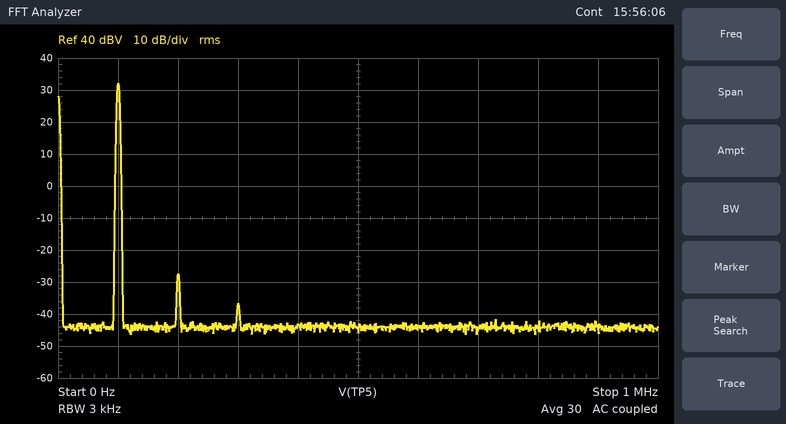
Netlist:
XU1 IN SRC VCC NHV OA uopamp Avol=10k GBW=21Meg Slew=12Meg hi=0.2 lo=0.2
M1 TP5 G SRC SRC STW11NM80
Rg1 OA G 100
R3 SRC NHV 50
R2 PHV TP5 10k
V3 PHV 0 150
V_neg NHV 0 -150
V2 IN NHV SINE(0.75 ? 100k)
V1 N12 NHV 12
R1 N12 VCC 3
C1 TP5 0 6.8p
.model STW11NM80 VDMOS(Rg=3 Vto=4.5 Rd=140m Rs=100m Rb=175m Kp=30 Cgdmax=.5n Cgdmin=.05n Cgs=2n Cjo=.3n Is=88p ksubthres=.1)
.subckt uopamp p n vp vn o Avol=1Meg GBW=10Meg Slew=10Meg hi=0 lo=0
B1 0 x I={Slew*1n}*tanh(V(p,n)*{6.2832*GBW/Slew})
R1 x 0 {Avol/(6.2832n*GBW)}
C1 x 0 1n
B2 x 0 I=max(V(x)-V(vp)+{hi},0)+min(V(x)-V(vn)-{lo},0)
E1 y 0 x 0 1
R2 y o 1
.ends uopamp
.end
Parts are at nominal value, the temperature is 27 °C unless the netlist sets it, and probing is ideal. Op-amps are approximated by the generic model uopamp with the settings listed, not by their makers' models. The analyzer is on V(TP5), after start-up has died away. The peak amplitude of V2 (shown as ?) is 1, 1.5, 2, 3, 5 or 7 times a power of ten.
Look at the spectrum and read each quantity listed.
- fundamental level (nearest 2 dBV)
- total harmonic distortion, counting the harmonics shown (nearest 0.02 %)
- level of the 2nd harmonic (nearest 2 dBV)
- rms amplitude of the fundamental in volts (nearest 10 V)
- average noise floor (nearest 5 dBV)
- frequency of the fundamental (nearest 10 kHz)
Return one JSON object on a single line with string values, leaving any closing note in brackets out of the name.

{"fundamental level": "32 dBV", "total harmonic distortion, counting the harmonics shown": "0.10 %", "level of the 2nd harmonic": "-28 dBV", "rms amplitude of the fundamental in volts": "40 V", "average noise floor": "-45 dBV", "frequency of the fundamental": "100 kHz"}
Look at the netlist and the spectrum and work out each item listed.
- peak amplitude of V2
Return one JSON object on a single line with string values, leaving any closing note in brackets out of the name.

{"peak amplitude of V2": "300 mV"}
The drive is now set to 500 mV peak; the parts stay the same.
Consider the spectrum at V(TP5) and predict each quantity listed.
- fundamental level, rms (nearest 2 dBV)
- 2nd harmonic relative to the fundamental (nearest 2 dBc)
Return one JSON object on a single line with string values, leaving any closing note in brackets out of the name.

{"fundamental level, rms": "36 dBV", "2nd harmonic relative to the fundamental": "-54 dBc"}
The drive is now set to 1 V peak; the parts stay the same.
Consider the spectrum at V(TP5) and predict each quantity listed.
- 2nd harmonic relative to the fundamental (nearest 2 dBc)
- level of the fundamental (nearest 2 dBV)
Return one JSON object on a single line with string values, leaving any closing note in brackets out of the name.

{"2nd harmonic relative to the fundamental": "-30 dBc", "level of the fundamental": "42 dBV"}
